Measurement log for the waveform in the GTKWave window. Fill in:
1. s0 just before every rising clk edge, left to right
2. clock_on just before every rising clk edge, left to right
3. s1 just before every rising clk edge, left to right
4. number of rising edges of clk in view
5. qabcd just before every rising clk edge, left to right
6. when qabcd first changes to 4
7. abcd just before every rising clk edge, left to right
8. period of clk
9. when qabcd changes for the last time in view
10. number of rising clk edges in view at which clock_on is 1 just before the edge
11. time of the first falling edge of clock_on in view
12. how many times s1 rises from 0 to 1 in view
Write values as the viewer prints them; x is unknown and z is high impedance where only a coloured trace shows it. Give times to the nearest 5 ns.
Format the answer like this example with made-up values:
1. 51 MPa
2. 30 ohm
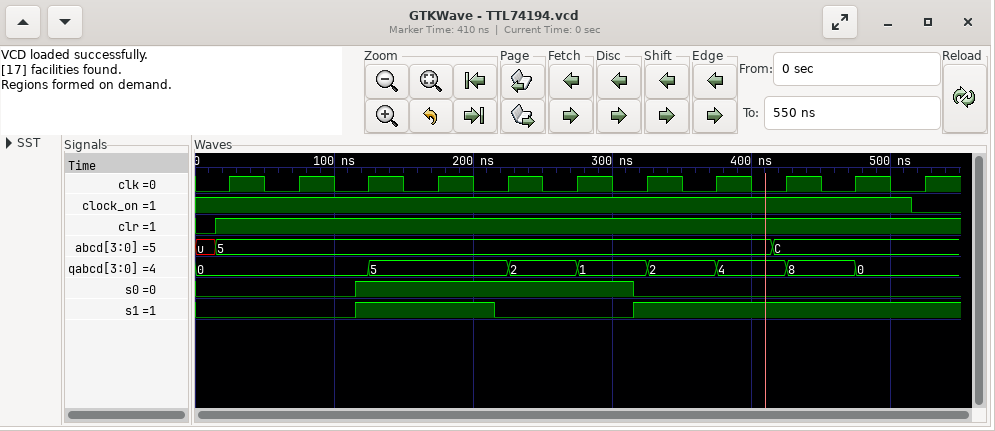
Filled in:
1. 0 0 1 1 1 1 0 0 0 0 0
2. 1 1 1 1 1 1 1 1 1 1 0
3. 0 0 1 1 0 0 1 1 1 1 1
4. 11
5. 0, 0, 0, 5, 5, 2, 1, 2, 4, 8, 0
6. 375 ns
7. 5, 5, 5, 5, 5, 5, 5, 5, C, C, C
8. 50 ns
9. 475 ns
10. 10
11. 515 ns
12. 2
